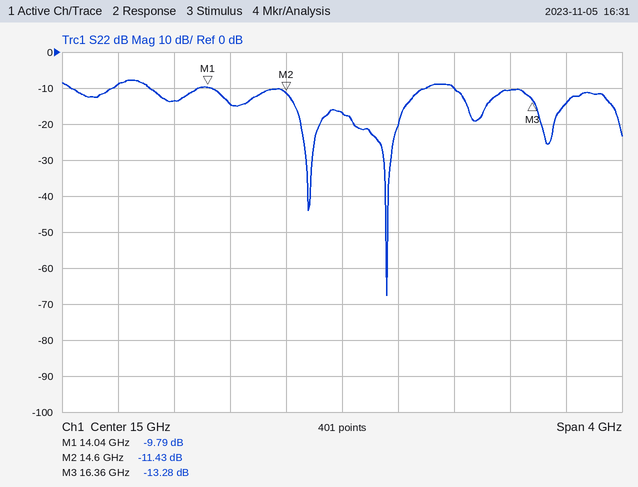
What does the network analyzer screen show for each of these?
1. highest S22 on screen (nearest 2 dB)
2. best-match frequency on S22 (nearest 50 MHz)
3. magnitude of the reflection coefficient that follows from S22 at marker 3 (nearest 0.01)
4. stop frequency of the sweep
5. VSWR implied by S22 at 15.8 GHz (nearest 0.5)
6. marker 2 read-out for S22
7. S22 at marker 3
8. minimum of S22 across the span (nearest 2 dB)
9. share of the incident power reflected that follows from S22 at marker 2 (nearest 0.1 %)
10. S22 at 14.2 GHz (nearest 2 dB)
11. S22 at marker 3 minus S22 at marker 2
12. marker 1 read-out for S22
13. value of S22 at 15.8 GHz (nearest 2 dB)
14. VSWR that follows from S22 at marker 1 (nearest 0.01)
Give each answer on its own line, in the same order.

-8 dB
15.30 GHz
0.22
17 GHz
2.0
-11.43 dB
-13.28 dB
-68 dB
7.2 %
-14 dB
-1.85 dB
-9.79 dB
-10 dB
1.96
